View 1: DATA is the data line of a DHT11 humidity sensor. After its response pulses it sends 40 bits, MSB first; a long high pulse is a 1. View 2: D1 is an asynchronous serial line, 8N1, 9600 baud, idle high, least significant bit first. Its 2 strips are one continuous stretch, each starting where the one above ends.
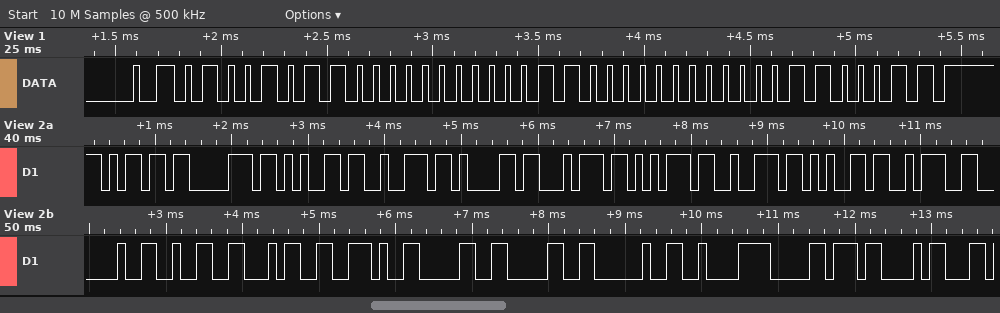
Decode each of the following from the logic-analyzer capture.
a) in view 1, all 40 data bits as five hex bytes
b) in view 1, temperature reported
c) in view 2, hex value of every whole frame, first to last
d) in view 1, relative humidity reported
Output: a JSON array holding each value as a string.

["4B 00 18 00 63", "24.0 °C", "6D 70 65 72 61 74 75 72 65 3A 20 32 34 2E 30 30 20 C2 B0 43", "75 %"]
